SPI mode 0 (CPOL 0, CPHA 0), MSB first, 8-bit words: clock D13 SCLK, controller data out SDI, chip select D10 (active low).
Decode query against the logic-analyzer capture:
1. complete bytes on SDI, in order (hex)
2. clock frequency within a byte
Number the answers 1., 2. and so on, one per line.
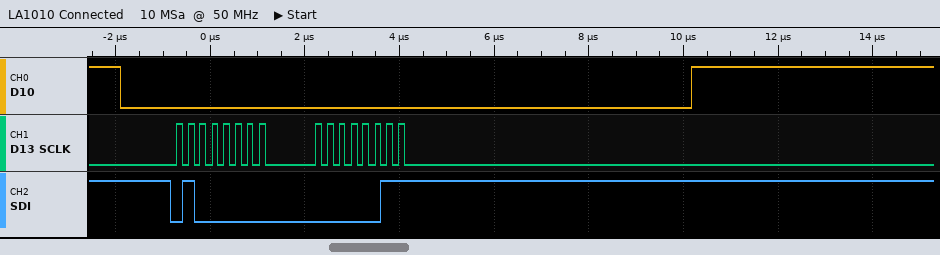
1. 40 03
2. 4 MHz
